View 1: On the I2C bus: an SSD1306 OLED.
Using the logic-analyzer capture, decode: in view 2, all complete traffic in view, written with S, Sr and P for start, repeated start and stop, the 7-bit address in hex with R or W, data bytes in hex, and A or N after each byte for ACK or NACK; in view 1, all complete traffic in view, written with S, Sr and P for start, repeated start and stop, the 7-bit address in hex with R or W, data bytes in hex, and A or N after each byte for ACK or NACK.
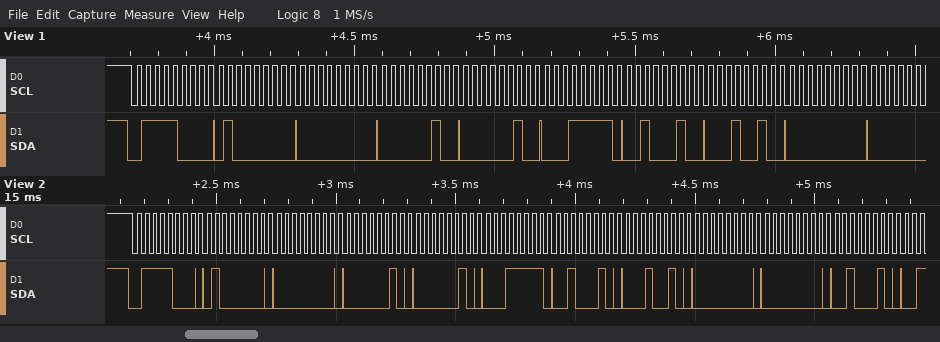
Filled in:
S 3CW A 40 A 00 A 02 A 02 A 1F A 22 A 12 A 00 A 00 A 22 A
S 3CW A 40 A 00 A 02 A 02 A 1F A 22 A 12 A 00 A
